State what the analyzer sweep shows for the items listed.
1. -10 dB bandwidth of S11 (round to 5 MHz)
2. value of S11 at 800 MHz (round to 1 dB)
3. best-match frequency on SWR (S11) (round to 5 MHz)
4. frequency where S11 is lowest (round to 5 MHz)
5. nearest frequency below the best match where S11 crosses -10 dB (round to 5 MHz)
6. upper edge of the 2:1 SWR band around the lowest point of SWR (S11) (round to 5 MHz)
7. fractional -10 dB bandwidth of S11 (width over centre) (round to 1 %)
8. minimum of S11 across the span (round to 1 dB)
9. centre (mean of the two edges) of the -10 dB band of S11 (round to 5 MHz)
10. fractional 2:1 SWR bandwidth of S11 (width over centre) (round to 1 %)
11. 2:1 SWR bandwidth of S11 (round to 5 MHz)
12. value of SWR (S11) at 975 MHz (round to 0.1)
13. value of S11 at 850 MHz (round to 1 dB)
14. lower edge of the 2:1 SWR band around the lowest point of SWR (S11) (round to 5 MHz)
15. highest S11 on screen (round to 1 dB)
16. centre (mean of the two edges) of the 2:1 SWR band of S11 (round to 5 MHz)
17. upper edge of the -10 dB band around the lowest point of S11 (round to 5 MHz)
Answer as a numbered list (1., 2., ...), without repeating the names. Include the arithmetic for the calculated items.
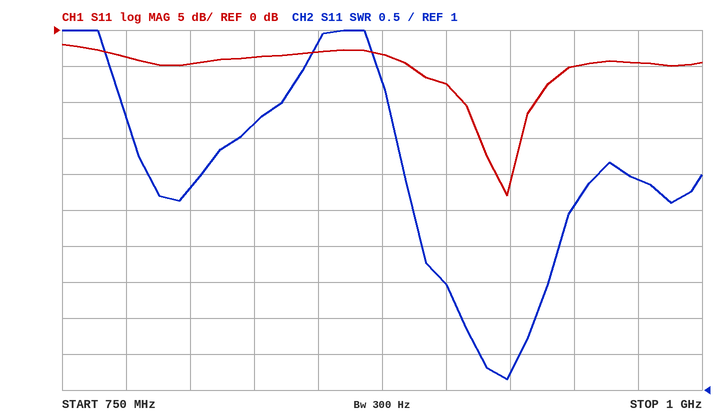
1. 935 MHz − 905 MHz = 30 MHz
2. -5 dB
3. 925 MHz
4. 925 MHz
5. 905 MHz
6. 935 MHz
7. 30 MHz / 920 MHz ≈ 3 %
8. -23 dB
9. 920 MHz
10. 30 MHz / 920 MHz ≈ 3 %
11. 935 MHz − 905 MHz = 30 MHz
12. 3.9
13. -3 dB
14. 905 MHz
15. -2 dB
16. 920 MHz
17. 935 MHz
